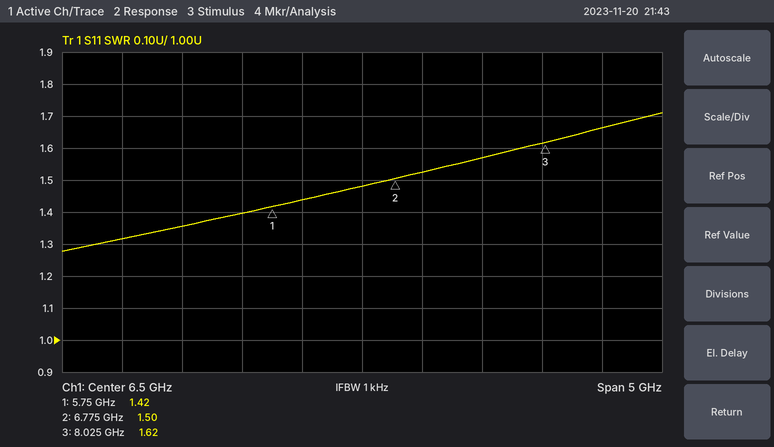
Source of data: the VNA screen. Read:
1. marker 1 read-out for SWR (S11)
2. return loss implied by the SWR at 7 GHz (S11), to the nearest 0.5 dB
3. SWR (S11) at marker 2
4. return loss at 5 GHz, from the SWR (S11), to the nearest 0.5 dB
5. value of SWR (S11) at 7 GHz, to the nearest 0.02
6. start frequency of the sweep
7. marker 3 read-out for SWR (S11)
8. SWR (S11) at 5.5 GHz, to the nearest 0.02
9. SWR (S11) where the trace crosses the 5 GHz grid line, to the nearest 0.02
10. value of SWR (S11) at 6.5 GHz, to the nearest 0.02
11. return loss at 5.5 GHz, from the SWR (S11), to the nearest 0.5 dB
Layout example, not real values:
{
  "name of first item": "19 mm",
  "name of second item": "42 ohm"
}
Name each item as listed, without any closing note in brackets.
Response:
{
  "marker 1 read-out for SWR": "1.42",
  "return loss implied by the SWR at 7 GHz (S11), to the nearest 0.5 dB": "13.5 dB",
  "SWR (S11) at marker 2": "1.50",
  "return loss at 5 GHz, from the SWR (S11), to the nearest 0.5 dB": "16.5 dB",
  "value of SWR (S11) at 7 GHz, to the nearest 0.02": "1.52",
  "start frequency of the sweep": "4 GHz",
  "marker 3 read-out for SWR": "1.62",
  "SWR (S11) at 5.5 GHz, to the nearest 0.02": "1.40",
  "SWR (S11) where the trace crosses the 5 GHz grid line, to the nearest 0.02": "1.36",
  "value of SWR (S11) at 6.5 GHz, to the nearest 0.02": "1.48",
  "return loss at 5.5 GHz, from the SWR (S11), to the nearest 0.5 dB": "15.5 dB"
}
